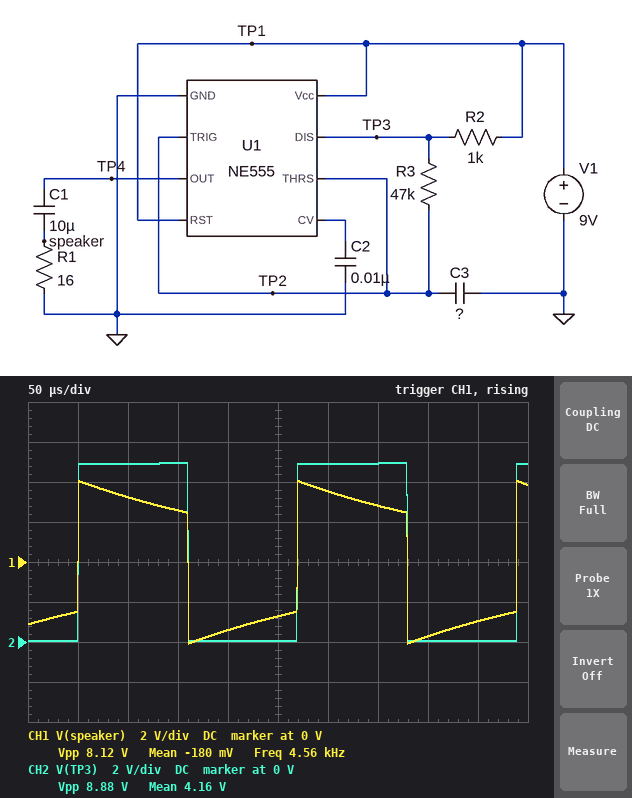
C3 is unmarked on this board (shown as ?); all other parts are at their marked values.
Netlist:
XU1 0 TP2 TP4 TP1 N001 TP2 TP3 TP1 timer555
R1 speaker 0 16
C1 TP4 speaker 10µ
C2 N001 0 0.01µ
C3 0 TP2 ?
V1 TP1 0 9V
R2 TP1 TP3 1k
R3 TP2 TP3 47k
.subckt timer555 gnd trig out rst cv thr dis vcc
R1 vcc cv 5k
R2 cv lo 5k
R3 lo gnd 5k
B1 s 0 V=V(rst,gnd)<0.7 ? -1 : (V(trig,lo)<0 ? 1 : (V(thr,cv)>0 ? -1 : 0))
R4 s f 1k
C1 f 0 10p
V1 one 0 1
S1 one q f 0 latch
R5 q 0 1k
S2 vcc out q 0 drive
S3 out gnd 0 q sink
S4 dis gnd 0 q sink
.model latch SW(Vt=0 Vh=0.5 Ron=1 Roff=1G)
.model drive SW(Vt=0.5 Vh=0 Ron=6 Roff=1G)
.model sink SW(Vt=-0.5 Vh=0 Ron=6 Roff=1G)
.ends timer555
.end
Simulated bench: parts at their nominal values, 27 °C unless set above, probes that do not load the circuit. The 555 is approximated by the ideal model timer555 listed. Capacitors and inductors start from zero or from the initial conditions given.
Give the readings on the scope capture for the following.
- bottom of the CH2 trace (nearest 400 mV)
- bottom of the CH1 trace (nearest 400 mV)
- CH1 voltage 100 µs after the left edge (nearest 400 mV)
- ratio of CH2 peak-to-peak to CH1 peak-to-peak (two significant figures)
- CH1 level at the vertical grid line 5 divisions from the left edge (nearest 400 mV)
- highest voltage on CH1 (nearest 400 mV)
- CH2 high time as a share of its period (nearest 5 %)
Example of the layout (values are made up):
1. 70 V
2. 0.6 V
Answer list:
1. 0 V
2. -4.0 V
3. 3.2 V
4. 1.1
5. -2.8 V
6. 4.0 V
7. 50 %
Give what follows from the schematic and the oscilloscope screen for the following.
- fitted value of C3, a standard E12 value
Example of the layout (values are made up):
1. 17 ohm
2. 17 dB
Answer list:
1. 3.3 nF
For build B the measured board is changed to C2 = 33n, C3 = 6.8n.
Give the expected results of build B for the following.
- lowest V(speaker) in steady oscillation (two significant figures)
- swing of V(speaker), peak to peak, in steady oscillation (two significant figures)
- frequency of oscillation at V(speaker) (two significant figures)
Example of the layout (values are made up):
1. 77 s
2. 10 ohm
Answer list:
1. -4.8 V
2. 9.6 V
3. 2.2 kHz
